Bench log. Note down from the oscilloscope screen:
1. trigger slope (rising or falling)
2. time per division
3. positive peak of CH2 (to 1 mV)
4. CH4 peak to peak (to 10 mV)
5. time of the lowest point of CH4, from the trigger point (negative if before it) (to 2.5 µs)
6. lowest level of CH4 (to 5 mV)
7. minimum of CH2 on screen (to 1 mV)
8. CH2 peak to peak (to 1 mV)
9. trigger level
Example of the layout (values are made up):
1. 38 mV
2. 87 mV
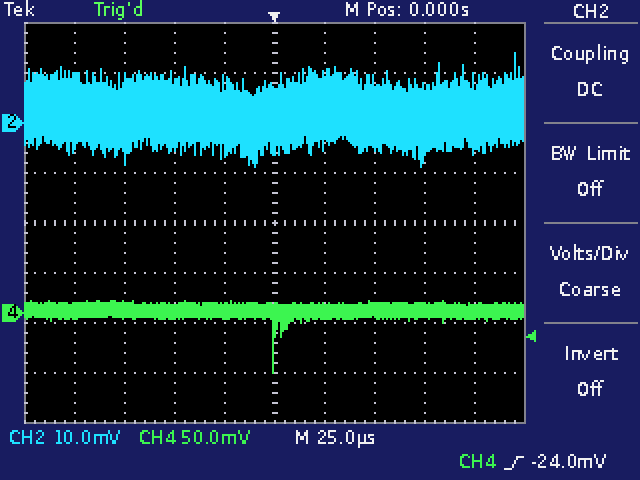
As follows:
1. rising
2. 25 µs
3. 14 mV
4. 70 mV
5. 0.0 µs
6. -60 mV
7. -9 mV
8. 23 mV
9. -24.0 mV
